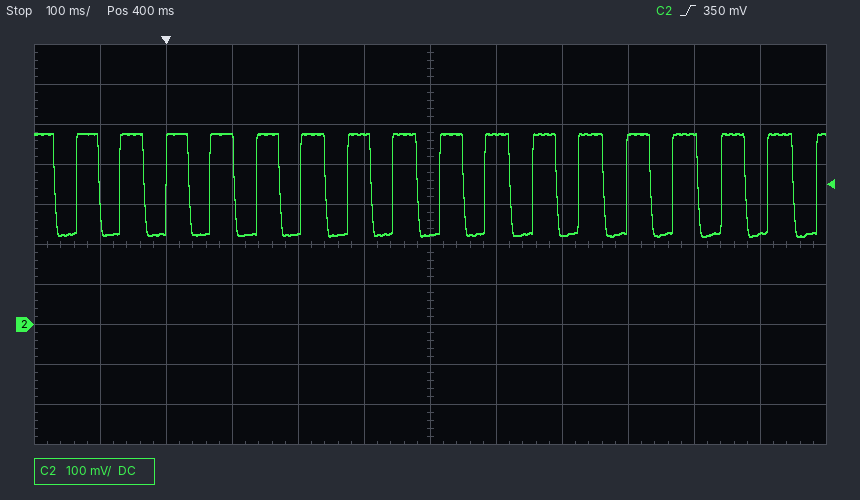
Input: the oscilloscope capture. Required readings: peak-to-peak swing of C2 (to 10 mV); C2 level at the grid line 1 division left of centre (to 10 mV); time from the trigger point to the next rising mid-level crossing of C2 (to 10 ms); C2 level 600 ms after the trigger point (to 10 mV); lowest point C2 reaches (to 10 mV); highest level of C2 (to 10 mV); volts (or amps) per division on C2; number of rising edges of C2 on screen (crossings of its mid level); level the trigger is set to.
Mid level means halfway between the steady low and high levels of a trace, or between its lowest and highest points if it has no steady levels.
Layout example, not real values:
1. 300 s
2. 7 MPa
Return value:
1. 260 mV
2. 480 mV
3. 70 ms
4. 230 mV
5. 220 mV
6. 480 mV
7. 100 mV
8. 17
9. 350 mV
